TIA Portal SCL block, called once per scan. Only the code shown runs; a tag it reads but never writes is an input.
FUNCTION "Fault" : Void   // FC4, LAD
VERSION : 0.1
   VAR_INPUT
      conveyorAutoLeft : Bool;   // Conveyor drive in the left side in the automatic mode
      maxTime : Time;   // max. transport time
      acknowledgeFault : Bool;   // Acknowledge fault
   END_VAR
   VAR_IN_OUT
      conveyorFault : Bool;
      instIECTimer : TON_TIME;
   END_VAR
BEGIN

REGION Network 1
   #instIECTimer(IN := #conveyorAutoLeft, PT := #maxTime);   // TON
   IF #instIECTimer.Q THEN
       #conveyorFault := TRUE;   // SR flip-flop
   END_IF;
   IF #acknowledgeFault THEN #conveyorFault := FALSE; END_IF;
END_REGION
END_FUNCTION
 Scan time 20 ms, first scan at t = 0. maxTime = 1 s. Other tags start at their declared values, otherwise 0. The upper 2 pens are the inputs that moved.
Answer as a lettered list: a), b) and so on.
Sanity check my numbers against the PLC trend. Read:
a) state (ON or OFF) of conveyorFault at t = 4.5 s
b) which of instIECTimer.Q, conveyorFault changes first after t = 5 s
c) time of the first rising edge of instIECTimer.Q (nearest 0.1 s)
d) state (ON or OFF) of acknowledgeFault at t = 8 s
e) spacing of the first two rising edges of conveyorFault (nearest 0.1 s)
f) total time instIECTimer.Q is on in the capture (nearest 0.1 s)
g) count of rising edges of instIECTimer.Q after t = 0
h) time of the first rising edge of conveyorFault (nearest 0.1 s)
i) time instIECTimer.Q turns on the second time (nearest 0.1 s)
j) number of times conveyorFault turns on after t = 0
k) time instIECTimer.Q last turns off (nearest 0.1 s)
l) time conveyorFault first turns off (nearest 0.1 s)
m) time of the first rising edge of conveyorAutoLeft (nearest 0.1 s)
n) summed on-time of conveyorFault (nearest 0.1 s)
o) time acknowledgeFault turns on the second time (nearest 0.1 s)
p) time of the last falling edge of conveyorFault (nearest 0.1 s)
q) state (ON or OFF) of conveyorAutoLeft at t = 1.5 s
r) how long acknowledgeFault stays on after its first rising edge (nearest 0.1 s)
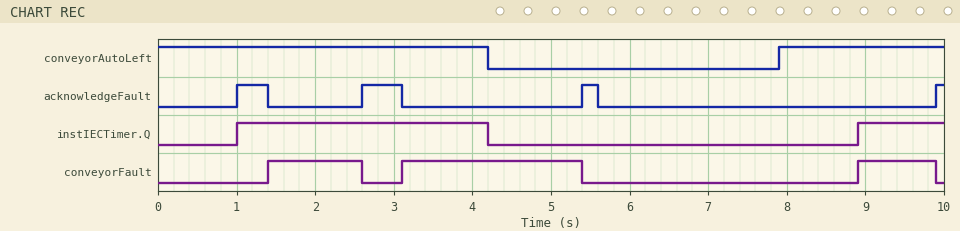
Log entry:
a) ON
b) conveyorFault
c) 1.0 s
d) OFF
e) 1.7 s
f) 4.3 s
g) 2
h) 1.4 s
i) 8.9 s
j) 3
k) 4.2 s
l) 2.6 s
m) 7.9 s
n) 4.5 s
o) 2.6 s
p) 9.9 s
q) ON
r) 0.4 s
